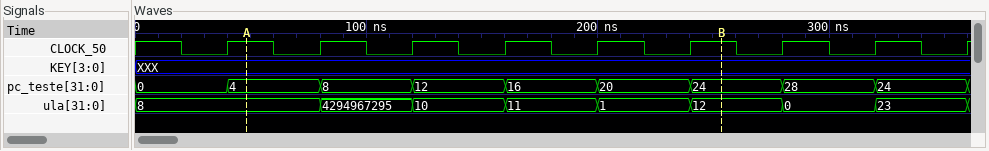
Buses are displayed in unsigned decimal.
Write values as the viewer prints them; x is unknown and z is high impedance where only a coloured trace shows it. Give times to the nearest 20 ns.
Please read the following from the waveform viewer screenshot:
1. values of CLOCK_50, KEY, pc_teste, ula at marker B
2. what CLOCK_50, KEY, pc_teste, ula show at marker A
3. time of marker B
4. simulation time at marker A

CLOCK_50=1, KEY=XXX, pc_teste=24, ula=12
CLOCK_50=1, KEY=XXX, pc_teste=4, ula=8
260 ns
40 ns
